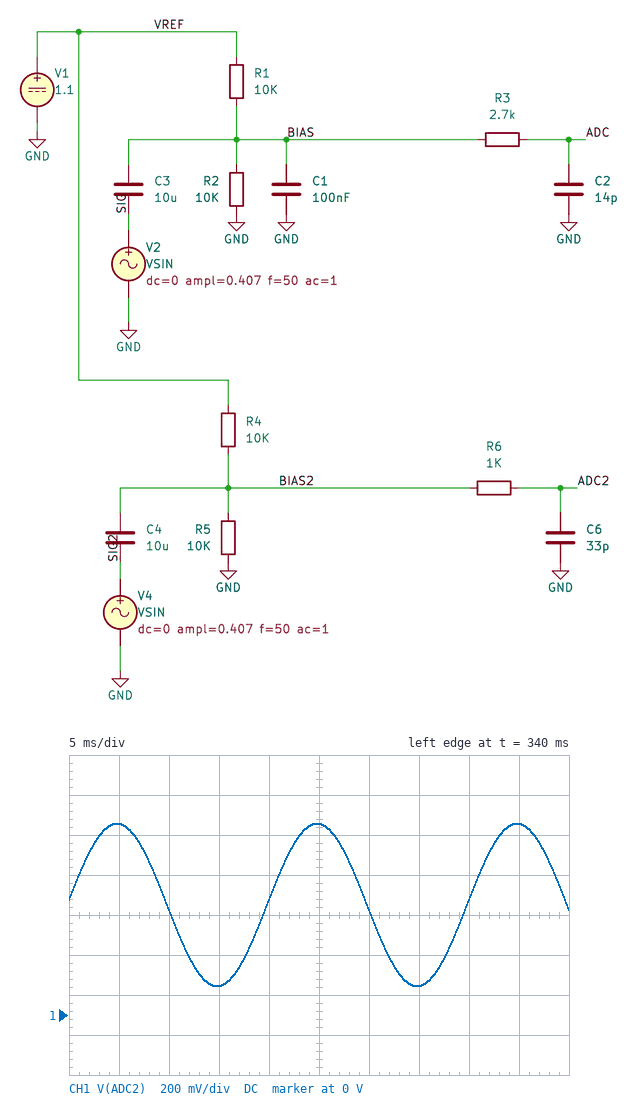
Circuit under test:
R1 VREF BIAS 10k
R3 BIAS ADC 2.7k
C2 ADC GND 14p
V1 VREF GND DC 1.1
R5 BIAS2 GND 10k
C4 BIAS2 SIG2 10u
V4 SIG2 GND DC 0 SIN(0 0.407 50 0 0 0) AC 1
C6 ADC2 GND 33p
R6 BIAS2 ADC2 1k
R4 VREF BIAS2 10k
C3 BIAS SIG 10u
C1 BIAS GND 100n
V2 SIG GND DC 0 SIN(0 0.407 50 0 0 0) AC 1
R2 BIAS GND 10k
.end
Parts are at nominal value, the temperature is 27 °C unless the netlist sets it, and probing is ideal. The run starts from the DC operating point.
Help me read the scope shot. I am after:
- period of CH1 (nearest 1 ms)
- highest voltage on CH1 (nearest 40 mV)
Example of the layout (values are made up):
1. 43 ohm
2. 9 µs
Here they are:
1. 20 ms
2. 960 mV
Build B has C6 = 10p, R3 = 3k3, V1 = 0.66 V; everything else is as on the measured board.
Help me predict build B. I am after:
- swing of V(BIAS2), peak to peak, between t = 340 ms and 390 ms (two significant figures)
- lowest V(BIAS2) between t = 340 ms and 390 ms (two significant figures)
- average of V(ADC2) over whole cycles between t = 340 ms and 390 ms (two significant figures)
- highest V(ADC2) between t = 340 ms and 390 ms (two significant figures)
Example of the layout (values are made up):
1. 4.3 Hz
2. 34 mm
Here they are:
1. 810 mV
2. -76 mV
3. 330 mV
4. 740 mV
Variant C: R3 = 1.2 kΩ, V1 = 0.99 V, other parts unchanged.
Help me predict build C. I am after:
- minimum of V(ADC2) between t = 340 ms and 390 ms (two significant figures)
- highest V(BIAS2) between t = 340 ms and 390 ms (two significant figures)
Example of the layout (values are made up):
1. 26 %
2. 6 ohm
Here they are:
1. 89 mV
2. 900 mV
